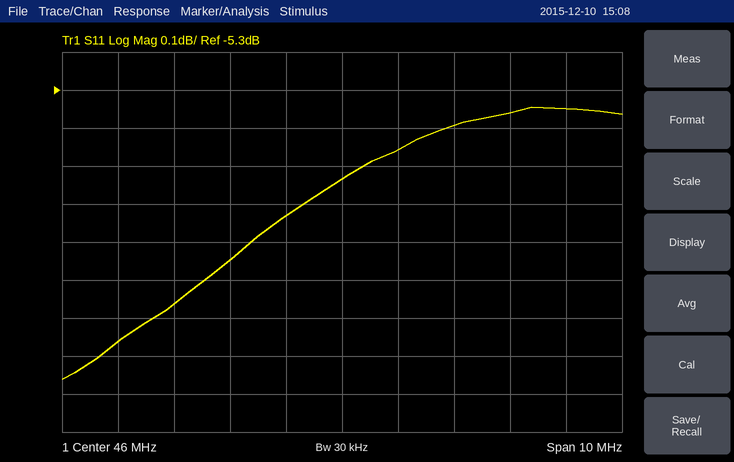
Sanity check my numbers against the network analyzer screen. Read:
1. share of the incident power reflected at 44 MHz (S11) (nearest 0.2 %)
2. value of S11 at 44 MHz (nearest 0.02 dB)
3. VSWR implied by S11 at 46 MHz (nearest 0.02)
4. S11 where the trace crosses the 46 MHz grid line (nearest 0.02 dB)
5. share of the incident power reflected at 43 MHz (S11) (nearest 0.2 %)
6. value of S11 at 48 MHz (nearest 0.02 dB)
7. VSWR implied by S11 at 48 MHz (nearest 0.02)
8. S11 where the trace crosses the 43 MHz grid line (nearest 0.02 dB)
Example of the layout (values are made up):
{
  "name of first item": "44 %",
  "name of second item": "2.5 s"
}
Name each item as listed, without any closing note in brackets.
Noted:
{
  "share of the incident power reflected at 44 MHz (S11)": "26.6 %",
  "value of S11 at 44 MHz": "-5.74 dB",
  "VSWR implied by S11 at 46 MHz": "3.24",
  "S11 where the trace crosses the 46 MHz grid line": "-5.54 dB",
  "share of the incident power reflected at 43 MHz (S11)": "26.0 %",
  "value of S11 at 48 MHz": "-5.40 dB",
  "VSWR implied by S11 at 48 MHz": "3.32",
  "S11 where the trace crosses the 43 MHz grid line": "-5.86 dB"
}
